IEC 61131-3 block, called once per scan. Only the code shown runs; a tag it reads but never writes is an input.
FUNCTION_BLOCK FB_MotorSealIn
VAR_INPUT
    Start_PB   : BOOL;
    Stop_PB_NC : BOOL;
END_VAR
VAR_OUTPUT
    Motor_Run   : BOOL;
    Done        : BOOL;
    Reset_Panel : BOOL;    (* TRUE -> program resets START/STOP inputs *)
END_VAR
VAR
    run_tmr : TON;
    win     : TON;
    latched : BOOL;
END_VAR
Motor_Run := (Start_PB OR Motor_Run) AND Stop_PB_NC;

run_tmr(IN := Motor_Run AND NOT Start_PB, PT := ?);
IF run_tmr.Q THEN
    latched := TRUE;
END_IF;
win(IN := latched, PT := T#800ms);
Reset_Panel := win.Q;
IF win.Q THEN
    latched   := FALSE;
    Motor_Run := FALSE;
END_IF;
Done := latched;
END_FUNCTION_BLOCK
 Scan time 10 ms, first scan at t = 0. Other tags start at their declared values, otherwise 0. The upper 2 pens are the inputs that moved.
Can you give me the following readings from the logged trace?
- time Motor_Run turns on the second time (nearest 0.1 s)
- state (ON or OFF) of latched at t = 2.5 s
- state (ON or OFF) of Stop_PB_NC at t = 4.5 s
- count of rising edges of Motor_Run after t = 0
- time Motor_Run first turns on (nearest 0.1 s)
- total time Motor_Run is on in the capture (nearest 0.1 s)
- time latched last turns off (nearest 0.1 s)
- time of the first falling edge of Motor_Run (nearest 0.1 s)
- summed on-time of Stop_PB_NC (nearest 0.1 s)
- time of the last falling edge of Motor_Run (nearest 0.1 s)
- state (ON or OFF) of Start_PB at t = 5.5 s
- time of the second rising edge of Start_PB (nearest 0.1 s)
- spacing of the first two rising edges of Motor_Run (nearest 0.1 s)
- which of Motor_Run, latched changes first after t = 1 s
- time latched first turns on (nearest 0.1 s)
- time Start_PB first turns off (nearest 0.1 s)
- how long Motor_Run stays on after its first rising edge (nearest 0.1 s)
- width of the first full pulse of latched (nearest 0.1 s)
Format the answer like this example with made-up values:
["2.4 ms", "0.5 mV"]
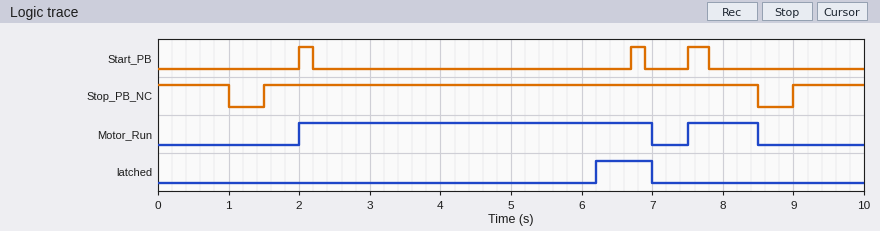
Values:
["7.5 s", "OFF", "ON", "2", "2.0 s", "6.0 s", "7.0 s", "7.0 s", "9.0 s", "8.5 s", "OFF", "6.7 s", "5.5 s", "Motor_Run", "6.2 s", "2.2 s", "5.0 s", "0.8 s"]
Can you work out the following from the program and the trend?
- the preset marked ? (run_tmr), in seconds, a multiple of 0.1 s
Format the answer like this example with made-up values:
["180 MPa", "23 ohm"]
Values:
["4.0 s"]
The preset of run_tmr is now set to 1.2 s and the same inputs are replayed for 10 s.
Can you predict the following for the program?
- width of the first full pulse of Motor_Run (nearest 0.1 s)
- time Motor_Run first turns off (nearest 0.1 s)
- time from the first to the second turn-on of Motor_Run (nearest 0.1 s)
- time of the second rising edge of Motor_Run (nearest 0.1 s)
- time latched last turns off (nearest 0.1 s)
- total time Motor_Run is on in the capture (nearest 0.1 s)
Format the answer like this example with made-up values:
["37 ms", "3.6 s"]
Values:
["2.2 s", "4.2 s", "4.7 s", "6.7 s", "4.2 s", "4.0 s"]
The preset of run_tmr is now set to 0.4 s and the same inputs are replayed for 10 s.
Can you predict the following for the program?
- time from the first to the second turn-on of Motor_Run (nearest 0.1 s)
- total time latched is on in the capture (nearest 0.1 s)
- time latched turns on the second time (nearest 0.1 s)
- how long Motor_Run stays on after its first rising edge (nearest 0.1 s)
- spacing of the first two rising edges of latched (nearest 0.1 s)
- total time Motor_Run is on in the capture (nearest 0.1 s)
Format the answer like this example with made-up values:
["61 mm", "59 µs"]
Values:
["4.7 s", "1.6 s", "7.3 s", "1.4 s", "4.7 s", "2.8 s"]
